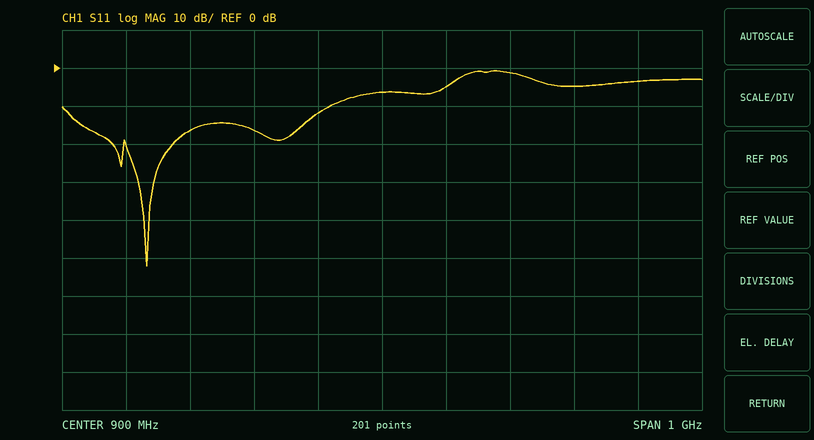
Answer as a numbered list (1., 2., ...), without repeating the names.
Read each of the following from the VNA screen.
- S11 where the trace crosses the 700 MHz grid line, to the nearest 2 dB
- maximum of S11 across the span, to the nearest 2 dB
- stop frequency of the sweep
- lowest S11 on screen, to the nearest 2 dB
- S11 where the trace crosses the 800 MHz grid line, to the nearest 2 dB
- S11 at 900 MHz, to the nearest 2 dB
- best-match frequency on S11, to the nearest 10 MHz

1. -16 dB
2. 0 dB
3. 1.4 GHz
4. -52 dB
5. -12 dB
6. -6 dB
7. 530 MHz
